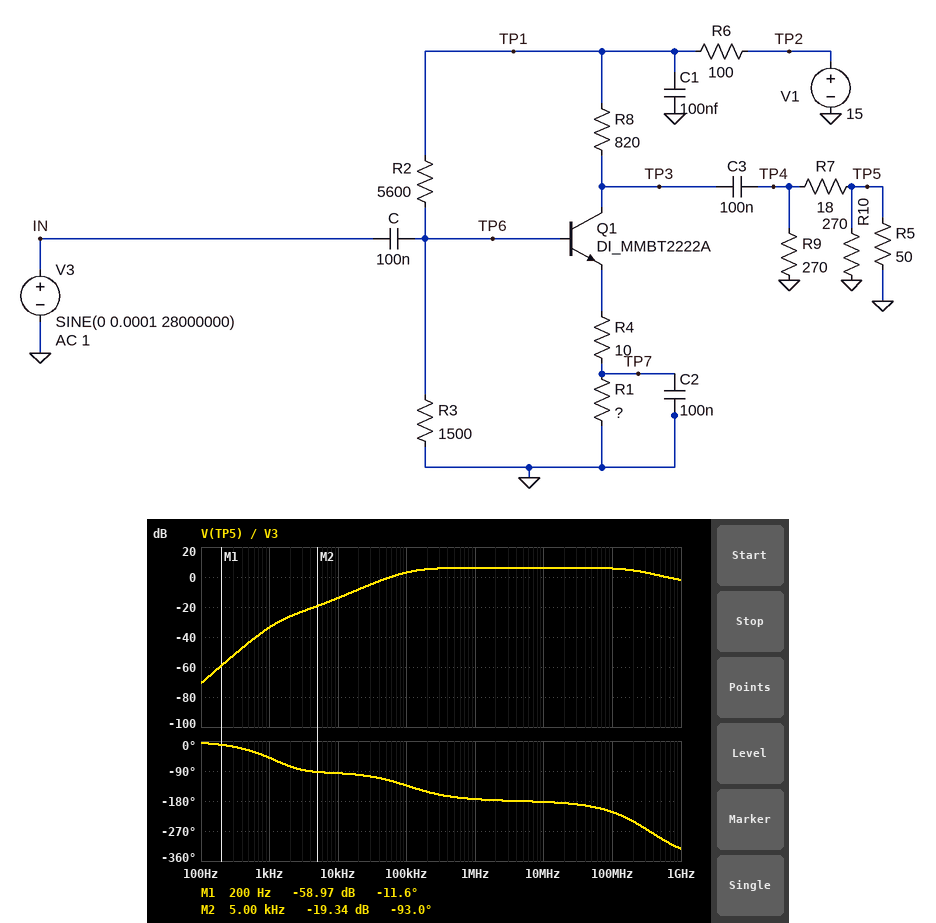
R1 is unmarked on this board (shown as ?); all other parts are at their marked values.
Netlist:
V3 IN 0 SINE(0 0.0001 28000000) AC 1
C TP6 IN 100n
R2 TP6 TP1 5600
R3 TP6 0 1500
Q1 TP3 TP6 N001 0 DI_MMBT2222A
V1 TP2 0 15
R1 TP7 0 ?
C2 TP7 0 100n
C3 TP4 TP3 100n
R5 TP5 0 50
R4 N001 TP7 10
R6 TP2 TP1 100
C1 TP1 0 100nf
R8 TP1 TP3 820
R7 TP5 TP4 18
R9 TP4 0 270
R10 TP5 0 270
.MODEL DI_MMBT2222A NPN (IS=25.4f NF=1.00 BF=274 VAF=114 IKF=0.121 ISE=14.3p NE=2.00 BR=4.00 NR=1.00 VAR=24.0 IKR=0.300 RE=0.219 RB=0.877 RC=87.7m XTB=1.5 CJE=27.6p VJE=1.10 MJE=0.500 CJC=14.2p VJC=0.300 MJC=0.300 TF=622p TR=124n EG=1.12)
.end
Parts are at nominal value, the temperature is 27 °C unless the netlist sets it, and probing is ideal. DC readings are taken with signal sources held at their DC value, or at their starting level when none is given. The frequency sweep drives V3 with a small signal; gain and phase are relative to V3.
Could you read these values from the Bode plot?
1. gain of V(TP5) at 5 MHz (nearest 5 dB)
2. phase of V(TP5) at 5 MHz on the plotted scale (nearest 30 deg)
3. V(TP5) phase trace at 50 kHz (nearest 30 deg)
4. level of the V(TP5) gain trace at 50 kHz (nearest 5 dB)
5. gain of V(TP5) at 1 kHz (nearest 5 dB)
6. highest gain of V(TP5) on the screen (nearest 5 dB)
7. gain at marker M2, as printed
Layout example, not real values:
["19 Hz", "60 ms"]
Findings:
["5 dB", "-180 deg", "-120 deg", "0 dB", "-35 dB", "5 dB", "-19.34 dB"]
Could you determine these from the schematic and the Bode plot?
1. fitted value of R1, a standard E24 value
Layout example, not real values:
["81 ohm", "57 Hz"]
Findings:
["470 Ω"]
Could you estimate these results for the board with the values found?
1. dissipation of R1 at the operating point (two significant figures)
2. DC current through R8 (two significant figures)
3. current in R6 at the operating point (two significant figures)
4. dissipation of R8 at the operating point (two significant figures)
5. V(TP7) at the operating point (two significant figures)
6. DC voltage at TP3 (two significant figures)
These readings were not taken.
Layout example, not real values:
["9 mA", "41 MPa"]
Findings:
["11 mW", "4.8 mA", "6.8 mA", "19 mW", "2.3 V", "10 V"]
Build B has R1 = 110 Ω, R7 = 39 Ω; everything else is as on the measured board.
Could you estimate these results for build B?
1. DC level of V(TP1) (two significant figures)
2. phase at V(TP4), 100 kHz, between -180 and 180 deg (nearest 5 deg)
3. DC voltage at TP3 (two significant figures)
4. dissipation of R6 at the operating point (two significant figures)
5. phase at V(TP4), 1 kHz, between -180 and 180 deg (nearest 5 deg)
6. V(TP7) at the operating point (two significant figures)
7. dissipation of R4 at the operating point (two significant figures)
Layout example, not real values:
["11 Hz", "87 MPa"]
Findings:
["13 V", "-115 deg", "1.8 V", "26 mW", "155 deg", "1.6 V", "2.1 mW"]
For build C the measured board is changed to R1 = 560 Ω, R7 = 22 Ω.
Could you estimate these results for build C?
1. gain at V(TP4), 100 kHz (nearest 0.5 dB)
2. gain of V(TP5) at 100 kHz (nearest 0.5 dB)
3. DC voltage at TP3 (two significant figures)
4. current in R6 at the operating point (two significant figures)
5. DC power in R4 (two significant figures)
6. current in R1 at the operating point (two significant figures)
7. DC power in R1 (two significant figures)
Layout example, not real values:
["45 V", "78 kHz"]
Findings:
["6.5 dB", "2.5 dB", "11 V", "6.1 mA", "170 µW", "4.1 mA", "9.5 mW"]
